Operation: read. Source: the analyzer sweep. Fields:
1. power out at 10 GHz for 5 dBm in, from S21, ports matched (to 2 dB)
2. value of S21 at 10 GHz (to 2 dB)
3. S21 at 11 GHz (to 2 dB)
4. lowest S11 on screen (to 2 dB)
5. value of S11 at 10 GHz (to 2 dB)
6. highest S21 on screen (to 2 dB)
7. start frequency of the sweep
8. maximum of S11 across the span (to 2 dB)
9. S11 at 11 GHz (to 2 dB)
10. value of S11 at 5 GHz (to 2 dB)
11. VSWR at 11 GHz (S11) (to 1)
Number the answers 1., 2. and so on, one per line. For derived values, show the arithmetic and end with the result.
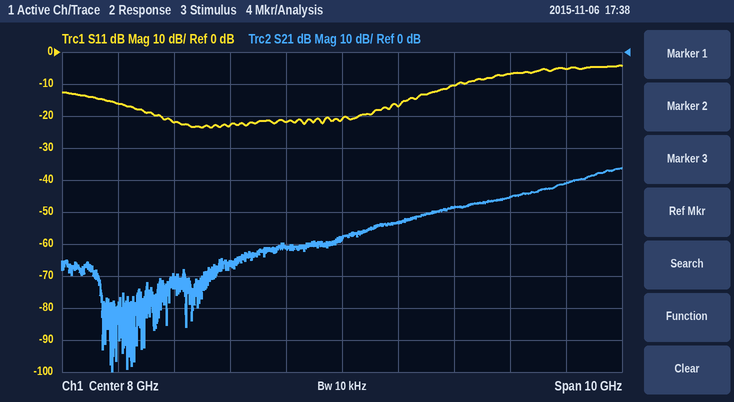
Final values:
1. 5 dBm + (-48 dB) = -44 dBm
2. -48 dB
3. -46 dB
4. -24 dB
5. -10 dB
6. -36 dB
7. 3 GHz
8. -4 dB
9. -6 dB
10. -22 dB
11. |Γ| = 10^(-6/20) = 0.5012; VSWR = (1 + 0.5012)/(1 − 0.5012) ≈ 3
